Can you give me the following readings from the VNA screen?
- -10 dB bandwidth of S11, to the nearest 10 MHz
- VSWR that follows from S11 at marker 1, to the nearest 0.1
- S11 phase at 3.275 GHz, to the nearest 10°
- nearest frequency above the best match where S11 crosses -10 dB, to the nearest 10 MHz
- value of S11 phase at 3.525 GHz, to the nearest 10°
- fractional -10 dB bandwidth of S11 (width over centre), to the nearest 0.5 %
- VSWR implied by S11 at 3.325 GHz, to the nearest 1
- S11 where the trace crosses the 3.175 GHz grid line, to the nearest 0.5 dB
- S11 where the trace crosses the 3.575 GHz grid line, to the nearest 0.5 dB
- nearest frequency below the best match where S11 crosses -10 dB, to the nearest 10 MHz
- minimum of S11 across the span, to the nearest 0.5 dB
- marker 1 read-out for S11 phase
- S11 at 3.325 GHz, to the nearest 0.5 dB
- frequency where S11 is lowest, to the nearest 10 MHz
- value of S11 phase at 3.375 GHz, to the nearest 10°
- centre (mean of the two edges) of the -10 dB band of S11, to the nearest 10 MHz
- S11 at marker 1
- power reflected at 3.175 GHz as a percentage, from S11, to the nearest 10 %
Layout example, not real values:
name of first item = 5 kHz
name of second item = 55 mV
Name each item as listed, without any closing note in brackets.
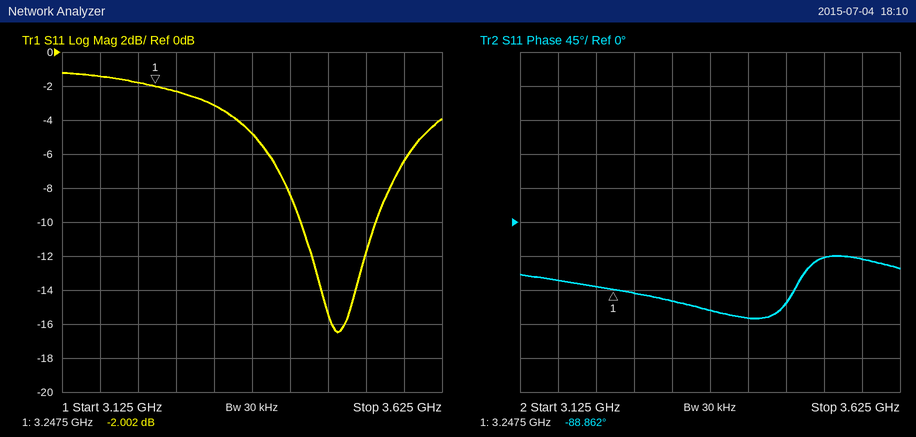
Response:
-10 dB bandwidth of S11, to the nearest 10 MHz = 100 MHz
VSWR that follows from S11 at marker 1, to the nearest 0.1 = 8.7
S11 phase at 3.275 GHz, to the nearest 10° = -90°
nearest frequency above the best match where S11 crosses -10 dB, to the nearest 10 MHz = 3.54 GHz
value of S11 phase at 3.525 GHz, to the nearest 10° = -50°
fractional -10 dB bandwidth of S11 (width over centre), to the nearest 0.5 % = 3.0 %
VSWR implied by S11 at 3.325 GHz, to the nearest 1 = 6
S11 where the trace crosses the 3.175 GHz grid line, to the nearest 0.5 dB = -1.5 dB
S11 where the trace crosses the 3.575 GHz grid line, to the nearest 0.5 dB = -6.5 dB
nearest frequency below the best match where S11 crosses -10 dB, to the nearest 10 MHz = 3.44 GHz
minimum of S11 across the span, to the nearest 0.5 dB = -16.5 dB
marker 1 read-out for S11 phase = -88.862°
S11 at 3.325 GHz, to the nearest 0.5 dB = -3.0 dB
frequency where S11 is lowest, to the nearest 10 MHz = 3.49 GHz
value of S11 phase at 3.375 GHz, to the nearest 10° = -120°
centre (mean of the two edges) of the -10 dB band of S11, to the nearest 10 MHz = 3.49 GHz
S11 at marker 1 = -2.002 dB
power reflected at 3.175 GHz as a percentage, from S11, to the nearest 10 % = 70 %
